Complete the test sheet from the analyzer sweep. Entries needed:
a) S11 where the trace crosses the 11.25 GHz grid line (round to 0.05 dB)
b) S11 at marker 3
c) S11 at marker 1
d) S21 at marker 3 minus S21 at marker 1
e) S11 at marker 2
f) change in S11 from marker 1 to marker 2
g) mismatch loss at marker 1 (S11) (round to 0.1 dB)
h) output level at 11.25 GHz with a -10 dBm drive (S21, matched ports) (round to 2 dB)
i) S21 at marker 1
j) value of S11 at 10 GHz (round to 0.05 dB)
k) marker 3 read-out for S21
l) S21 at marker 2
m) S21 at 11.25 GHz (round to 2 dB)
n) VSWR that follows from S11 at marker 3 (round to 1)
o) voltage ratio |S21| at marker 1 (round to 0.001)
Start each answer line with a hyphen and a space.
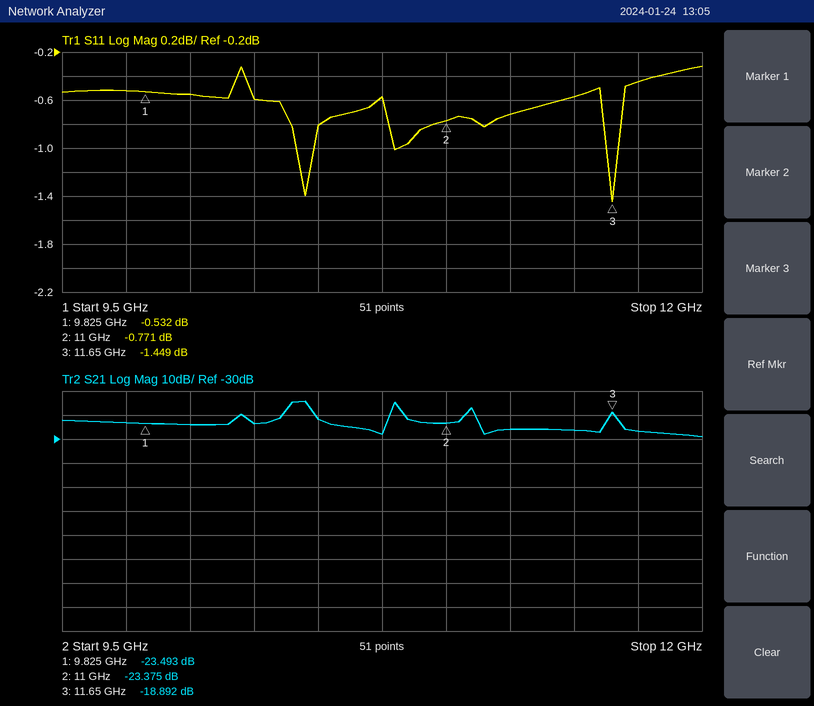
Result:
- -0.70 dB
- -1.449 dB
- -0.532 dB
- 4.601 dB
- -0.771 dB
- -0.239 dB
- 9.4 dB
- -36 dBm
- -23.493 dB
- -0.55 dB
- -18.892 dB
- -23.375 dB
- -26 dB
- 12
- 0.067
